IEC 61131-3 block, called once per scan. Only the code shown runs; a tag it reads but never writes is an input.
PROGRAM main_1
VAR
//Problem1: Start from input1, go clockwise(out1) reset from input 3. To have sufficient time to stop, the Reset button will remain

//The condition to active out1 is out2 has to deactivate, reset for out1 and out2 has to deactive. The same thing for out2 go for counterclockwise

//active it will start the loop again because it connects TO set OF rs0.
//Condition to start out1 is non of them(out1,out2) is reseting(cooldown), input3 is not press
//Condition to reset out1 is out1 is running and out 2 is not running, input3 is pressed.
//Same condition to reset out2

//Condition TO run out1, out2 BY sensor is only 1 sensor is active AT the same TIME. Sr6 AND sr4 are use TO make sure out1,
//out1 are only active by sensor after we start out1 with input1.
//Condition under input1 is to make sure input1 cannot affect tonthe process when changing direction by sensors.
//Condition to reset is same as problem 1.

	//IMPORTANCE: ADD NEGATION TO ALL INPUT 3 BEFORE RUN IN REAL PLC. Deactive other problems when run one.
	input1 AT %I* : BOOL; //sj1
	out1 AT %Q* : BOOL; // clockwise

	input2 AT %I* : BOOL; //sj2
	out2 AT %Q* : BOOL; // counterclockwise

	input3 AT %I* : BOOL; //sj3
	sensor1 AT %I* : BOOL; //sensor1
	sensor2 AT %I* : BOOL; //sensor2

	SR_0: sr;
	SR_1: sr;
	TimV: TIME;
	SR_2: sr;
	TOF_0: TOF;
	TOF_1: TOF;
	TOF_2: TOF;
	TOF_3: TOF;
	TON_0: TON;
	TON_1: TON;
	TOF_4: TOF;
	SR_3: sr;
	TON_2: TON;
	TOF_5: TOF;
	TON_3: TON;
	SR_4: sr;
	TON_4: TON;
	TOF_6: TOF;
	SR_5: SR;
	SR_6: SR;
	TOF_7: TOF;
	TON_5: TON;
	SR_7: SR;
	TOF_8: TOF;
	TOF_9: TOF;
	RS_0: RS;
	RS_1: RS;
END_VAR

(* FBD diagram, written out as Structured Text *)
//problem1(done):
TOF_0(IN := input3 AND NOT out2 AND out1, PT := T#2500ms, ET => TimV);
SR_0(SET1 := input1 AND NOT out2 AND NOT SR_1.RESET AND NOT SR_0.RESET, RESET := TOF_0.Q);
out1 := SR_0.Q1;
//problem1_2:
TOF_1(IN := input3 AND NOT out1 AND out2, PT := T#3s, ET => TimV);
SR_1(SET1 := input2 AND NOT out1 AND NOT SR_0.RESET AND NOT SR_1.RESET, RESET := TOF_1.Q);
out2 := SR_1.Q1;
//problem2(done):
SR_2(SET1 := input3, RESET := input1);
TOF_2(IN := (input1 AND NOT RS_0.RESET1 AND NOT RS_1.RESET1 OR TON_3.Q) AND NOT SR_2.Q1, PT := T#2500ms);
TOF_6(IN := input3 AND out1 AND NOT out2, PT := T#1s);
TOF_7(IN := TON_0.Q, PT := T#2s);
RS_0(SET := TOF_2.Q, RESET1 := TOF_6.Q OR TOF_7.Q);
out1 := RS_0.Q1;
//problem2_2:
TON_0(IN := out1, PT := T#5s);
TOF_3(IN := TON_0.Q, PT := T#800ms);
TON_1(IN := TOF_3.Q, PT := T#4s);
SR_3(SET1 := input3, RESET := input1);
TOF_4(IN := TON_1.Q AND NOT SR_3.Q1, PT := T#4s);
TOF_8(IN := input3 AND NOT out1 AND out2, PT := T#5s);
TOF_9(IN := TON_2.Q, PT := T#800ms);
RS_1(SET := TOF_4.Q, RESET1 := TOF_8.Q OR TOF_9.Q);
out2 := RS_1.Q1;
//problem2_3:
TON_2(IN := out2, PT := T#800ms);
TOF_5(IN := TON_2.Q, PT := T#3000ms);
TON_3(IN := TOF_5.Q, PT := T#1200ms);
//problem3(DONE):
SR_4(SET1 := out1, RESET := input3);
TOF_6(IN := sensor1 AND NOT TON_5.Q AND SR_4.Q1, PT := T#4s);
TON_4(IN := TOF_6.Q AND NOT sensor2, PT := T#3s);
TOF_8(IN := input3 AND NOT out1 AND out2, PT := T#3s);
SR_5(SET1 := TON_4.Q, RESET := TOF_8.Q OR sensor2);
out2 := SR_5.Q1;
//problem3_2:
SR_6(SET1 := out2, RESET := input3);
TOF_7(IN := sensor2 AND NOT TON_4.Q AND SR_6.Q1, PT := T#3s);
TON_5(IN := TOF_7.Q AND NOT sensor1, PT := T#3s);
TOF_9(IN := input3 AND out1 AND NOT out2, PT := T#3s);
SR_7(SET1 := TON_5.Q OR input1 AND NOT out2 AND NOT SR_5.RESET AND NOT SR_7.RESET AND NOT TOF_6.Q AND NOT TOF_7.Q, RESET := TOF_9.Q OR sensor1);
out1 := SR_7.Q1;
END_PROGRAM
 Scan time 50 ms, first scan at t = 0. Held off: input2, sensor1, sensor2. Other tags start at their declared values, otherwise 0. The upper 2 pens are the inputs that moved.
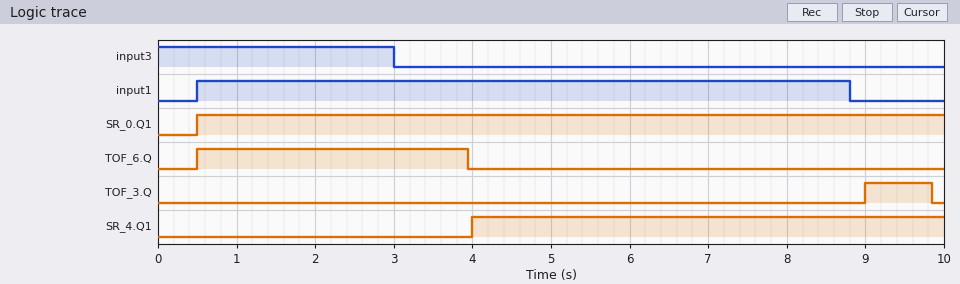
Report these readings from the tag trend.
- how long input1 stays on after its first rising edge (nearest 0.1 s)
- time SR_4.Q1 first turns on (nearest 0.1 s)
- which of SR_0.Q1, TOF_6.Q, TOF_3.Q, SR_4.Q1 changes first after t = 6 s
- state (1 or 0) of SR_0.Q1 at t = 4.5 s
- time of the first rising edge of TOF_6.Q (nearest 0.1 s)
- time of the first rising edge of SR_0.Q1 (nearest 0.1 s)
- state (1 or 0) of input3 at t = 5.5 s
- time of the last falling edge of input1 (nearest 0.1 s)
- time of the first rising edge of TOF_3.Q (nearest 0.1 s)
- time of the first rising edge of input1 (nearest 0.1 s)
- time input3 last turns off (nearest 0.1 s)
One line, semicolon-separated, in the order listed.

8.3 s; 4.0 s; TOF_3.Q; 1; 0.5 s; 0.5 s; 0; 8.8 s; 9.0 s; 0.5 s; 3.0 s
